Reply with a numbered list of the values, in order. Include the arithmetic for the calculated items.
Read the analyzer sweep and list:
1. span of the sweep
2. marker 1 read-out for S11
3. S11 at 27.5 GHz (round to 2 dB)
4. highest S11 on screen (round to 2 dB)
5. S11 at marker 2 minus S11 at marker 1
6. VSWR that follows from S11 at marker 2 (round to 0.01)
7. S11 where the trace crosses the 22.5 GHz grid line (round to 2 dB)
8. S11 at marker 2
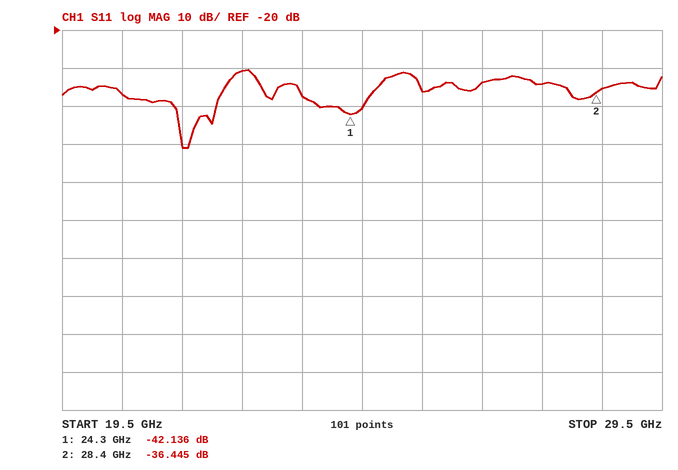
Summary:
1. 10 GHz
2. -42.136 dB
3. -34 dB
4. -30 dB
5. -36.445 − (-42.136) = 5.691 dB
6. (1 + 0.0151)/(1 − 0.0151) ≈ 1.03
7. -30 dB
8. -36.445 dB
